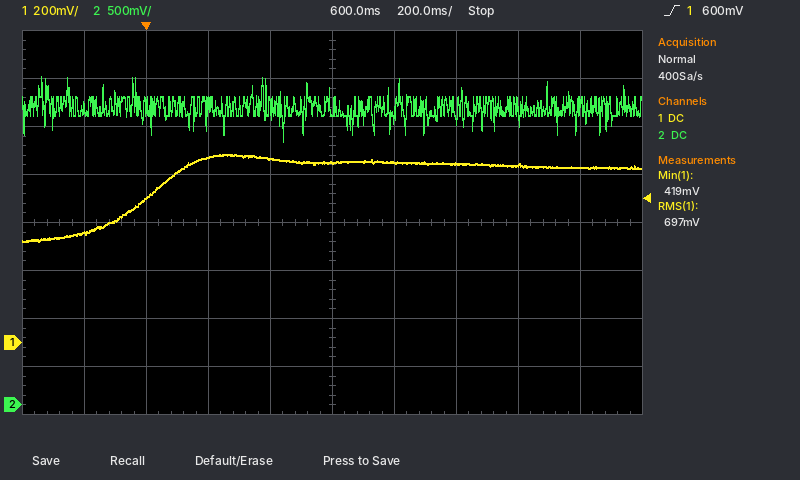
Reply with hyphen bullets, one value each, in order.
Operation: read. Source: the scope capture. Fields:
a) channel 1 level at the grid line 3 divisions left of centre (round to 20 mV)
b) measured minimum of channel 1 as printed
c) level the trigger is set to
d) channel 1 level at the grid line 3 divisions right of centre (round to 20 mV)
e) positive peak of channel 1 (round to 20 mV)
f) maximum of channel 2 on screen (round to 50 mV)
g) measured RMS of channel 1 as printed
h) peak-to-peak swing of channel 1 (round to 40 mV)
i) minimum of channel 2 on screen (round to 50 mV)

- 600 mV
- 419 mV
- 600 mV
- 740 mV
- 780 mV
- 3.40 V
- 697 mV
- 360 mV
- 2.75 V
